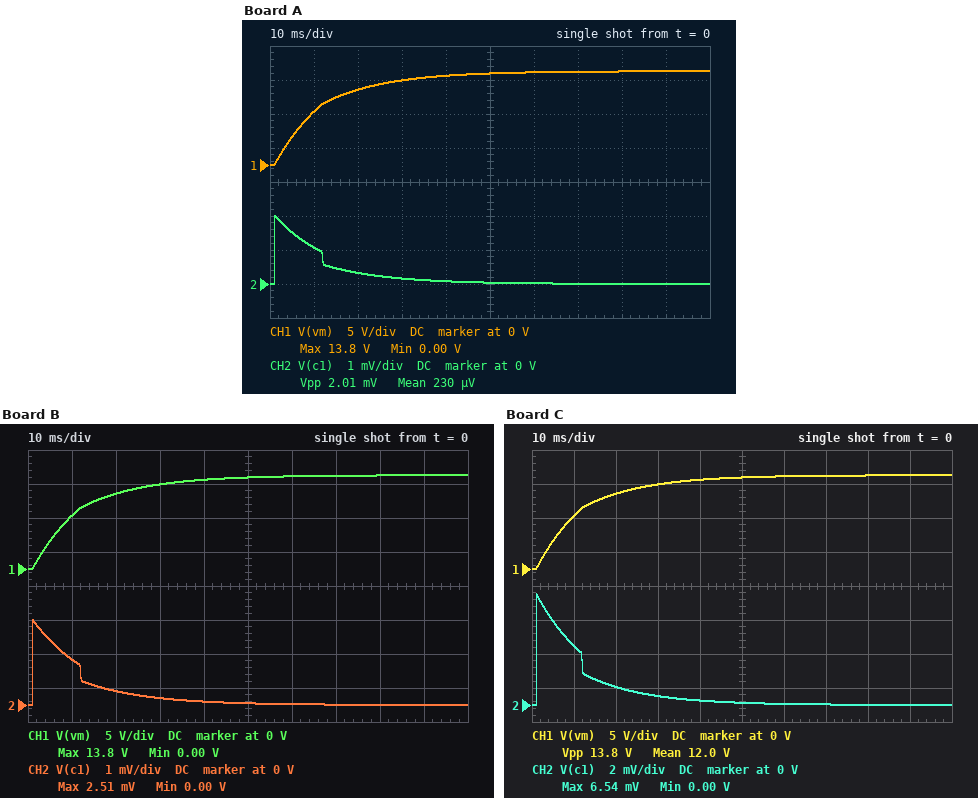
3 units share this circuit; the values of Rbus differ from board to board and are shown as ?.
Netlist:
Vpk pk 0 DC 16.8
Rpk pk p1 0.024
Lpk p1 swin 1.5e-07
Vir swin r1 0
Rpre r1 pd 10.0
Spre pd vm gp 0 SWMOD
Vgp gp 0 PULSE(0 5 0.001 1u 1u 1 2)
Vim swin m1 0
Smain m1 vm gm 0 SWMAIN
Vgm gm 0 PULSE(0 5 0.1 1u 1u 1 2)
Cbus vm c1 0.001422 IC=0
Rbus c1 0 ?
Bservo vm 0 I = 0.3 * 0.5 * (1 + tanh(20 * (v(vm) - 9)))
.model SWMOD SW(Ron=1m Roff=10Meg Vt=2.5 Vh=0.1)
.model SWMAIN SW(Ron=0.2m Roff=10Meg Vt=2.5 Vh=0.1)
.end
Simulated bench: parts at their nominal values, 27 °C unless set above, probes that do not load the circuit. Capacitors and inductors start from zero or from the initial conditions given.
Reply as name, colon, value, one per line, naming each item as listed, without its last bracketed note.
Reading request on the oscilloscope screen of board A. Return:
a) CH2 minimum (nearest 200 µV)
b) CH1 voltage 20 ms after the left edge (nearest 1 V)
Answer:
CH2 minimum: 0 V
CH1 voltage 20 ms after the left edge: 11 V
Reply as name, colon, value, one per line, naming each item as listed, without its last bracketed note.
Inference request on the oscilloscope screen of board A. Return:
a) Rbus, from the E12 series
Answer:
Rbus, from the E12 series: 1.2 mΩ
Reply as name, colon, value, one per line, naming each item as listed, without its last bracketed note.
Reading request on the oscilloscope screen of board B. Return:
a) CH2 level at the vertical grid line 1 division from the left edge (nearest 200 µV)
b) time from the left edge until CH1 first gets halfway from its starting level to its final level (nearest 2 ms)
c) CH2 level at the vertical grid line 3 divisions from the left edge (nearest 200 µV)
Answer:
CH2 level at the vertical grid line 1 division from the left edge: 1.4 mV
time from the left edge until CH1 first gets halfway from its starting level to its final level: 8 ms
CH2 level at the vertical grid line 3 divisions from the left edge: 200 µV
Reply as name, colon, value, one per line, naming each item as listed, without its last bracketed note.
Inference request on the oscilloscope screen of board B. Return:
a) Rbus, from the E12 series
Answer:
Rbus, from the E12 series: 1.5 mΩ
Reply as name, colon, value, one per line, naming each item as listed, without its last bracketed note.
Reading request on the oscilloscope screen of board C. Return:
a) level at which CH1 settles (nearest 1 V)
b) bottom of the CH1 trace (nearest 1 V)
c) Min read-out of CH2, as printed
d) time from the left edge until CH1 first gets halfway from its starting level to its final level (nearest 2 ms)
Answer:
level at which CH1 settles: 14 V
bottom of the CH1 trace: 0 V
Min read-out of CH2, as printed: 0.00 V
time from the left edge until CH1 first gets halfway from its starting level to its final level: 8 ms
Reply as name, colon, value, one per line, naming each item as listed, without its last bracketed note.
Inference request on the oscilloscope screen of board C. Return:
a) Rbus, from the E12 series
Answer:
Rbus, from the E12 series: 3.9 mΩ
